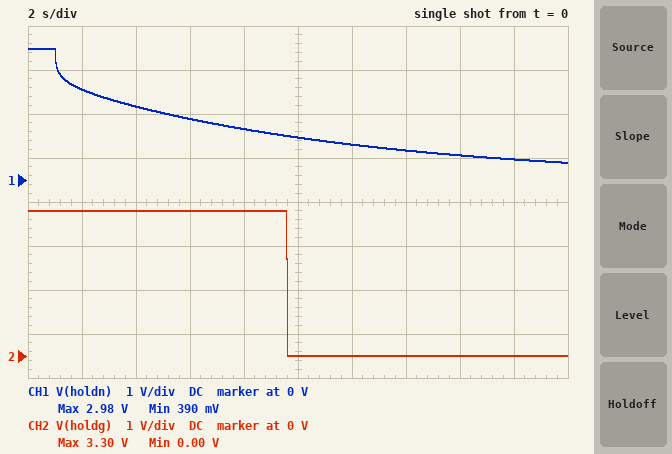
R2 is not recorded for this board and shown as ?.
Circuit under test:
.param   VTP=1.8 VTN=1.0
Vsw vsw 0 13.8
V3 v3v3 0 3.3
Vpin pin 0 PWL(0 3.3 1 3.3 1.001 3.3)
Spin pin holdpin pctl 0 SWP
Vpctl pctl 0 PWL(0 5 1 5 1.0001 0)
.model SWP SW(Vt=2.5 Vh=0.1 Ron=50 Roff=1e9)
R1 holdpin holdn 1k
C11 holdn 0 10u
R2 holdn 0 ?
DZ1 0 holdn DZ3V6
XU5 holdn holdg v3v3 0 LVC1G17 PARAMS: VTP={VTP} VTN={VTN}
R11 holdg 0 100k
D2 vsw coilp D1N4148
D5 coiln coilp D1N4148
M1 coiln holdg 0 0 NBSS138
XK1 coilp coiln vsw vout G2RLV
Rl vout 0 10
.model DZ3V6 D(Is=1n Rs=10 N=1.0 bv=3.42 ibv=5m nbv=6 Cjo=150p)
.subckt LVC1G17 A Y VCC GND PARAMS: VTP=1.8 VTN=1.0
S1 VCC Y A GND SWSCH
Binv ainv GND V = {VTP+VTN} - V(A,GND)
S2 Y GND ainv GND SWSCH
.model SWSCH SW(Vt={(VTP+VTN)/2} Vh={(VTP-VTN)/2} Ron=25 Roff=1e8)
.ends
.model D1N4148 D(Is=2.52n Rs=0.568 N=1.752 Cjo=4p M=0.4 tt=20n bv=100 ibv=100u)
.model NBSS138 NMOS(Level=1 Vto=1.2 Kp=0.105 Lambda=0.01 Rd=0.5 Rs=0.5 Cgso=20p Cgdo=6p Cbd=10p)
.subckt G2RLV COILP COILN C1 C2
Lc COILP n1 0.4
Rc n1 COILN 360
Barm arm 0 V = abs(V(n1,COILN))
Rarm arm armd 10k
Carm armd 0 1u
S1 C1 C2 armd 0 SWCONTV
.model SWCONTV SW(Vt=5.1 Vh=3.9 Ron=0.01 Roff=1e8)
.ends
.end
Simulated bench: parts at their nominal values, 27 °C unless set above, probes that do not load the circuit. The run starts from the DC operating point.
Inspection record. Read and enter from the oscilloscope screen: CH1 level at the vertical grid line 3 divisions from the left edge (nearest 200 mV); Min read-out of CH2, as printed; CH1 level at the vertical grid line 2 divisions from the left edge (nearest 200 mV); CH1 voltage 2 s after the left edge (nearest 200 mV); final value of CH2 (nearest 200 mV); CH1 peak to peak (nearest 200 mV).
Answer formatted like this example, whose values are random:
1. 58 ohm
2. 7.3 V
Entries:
1. 1.4 V
2. 0.00 V
3. 1.6 V
4. 2.0 V
5. 0 V
6. 2.6 V
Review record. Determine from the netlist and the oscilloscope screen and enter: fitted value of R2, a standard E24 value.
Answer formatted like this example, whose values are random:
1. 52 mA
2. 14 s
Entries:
1. 1.1 MΩ
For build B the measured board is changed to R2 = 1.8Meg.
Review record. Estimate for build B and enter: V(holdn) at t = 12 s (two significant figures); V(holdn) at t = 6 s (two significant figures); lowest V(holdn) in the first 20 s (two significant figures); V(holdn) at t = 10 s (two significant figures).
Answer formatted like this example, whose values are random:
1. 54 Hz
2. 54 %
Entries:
1. 1.1 V
2. 1.6 V
3. 730 mV
4. 1.3 V
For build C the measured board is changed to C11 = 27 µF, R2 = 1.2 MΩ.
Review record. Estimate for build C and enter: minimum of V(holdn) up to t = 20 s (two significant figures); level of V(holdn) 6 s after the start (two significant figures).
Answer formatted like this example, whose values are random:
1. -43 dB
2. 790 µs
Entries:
1. 1.2 V
2. 1.9 V
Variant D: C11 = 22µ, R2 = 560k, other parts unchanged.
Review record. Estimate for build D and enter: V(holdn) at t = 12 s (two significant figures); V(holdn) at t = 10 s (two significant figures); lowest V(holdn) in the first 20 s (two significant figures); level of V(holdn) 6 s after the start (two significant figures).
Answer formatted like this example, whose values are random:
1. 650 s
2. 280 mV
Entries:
1. 940 mV
2. 1.1 V
3. 490 mV
4. 1.5 V
